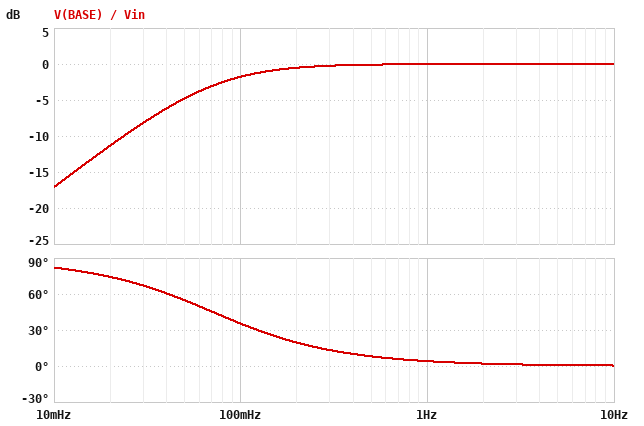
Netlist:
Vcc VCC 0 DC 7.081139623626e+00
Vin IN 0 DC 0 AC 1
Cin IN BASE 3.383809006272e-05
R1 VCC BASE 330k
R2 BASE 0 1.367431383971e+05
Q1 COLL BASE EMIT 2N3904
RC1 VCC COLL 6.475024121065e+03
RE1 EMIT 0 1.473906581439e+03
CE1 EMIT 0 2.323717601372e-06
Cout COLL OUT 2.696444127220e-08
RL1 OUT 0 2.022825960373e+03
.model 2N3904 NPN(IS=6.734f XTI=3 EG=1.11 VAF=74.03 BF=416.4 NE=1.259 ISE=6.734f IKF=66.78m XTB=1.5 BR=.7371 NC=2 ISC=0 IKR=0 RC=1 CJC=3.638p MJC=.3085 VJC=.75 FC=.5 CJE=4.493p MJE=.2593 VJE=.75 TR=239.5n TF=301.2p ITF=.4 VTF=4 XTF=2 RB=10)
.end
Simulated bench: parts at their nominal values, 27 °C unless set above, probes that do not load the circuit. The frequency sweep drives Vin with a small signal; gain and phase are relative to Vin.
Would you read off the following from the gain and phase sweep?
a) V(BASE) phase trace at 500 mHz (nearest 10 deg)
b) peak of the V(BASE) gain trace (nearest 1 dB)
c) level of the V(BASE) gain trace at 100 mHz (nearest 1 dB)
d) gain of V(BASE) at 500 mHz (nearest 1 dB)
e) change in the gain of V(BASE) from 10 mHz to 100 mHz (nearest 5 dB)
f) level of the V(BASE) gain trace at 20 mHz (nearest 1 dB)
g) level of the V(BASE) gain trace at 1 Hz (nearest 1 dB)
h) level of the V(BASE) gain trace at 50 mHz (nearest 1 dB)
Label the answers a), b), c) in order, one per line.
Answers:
a) 10 deg
b) 0 dB
c) -2 dB
d) 0 dB
e) 15 dB
f) -11 dB
g) 0 dB
h) -5 dB
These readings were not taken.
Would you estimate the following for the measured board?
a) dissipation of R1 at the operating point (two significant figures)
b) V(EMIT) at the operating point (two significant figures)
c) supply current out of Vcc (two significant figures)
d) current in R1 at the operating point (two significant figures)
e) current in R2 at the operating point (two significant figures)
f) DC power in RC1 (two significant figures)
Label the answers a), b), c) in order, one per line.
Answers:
a) 91 µW
b) 940 mV
c) 650 µA
d) 17 µA
e) 12 µA
f) 2.6 mW
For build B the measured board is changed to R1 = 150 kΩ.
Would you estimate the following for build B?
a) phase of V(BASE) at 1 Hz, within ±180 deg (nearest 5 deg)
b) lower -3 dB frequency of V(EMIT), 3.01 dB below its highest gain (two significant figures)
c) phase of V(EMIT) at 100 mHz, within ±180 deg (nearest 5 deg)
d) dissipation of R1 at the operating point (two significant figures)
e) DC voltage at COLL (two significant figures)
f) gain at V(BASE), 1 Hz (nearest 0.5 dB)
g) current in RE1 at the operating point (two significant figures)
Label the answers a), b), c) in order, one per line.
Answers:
a) 70 deg
b) 2.8 Hz
c) 90 deg
d) 170 µW
e) 1.4 V
f) -10.0 dB
g) 890 µA
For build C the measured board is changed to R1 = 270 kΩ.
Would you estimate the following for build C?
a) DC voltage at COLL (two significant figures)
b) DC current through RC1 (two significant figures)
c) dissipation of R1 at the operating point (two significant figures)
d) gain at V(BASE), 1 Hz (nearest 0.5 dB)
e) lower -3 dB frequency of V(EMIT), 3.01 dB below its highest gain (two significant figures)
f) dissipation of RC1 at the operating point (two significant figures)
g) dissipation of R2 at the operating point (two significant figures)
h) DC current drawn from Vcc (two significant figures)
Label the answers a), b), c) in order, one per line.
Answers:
a) 2.0 V
b) 790 µA
c) 100 µW
d) 0 dB
e) 74 mHz
f) 4.0 mW
g) 24 µW
h) 810 µA
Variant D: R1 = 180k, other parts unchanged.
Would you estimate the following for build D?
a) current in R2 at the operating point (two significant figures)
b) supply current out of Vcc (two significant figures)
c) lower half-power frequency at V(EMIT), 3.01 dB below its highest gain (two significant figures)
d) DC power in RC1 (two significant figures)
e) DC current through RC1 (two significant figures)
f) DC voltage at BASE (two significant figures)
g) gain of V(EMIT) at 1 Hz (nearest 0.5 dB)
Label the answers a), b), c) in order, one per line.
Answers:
a) 14 µA
b) 900 µA
c) 2.4 Hz
d) 4.9 mW
e) 870 µA
f) 2.0 V
g) -9.0 dB
